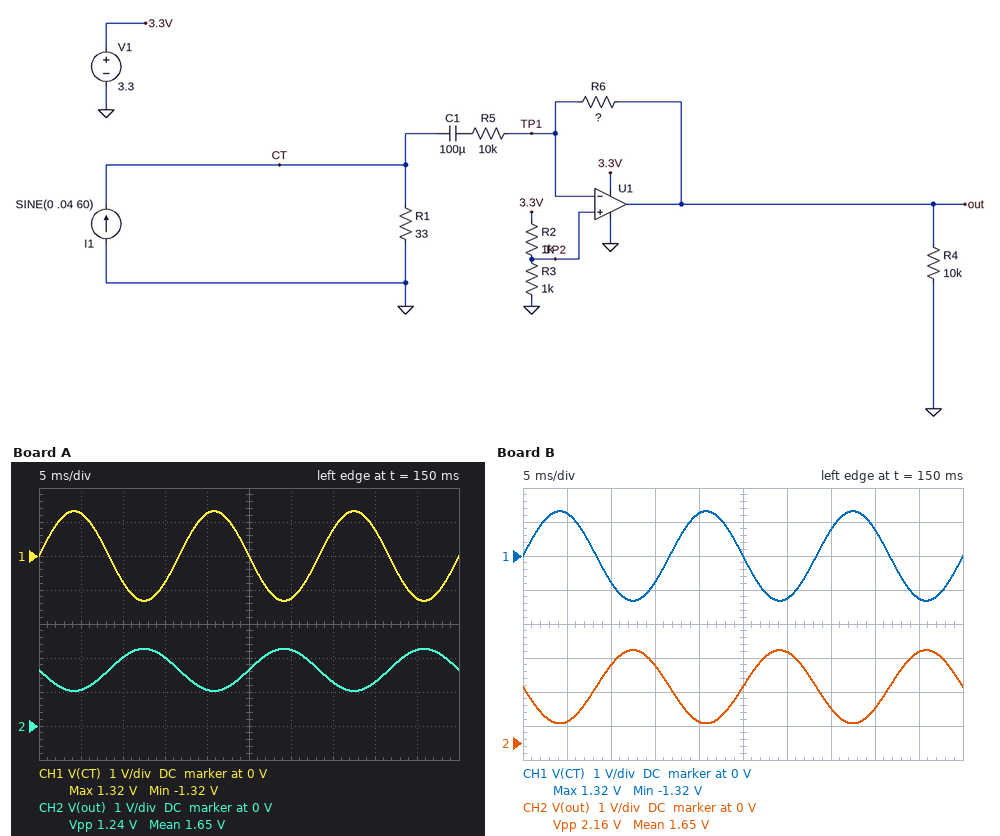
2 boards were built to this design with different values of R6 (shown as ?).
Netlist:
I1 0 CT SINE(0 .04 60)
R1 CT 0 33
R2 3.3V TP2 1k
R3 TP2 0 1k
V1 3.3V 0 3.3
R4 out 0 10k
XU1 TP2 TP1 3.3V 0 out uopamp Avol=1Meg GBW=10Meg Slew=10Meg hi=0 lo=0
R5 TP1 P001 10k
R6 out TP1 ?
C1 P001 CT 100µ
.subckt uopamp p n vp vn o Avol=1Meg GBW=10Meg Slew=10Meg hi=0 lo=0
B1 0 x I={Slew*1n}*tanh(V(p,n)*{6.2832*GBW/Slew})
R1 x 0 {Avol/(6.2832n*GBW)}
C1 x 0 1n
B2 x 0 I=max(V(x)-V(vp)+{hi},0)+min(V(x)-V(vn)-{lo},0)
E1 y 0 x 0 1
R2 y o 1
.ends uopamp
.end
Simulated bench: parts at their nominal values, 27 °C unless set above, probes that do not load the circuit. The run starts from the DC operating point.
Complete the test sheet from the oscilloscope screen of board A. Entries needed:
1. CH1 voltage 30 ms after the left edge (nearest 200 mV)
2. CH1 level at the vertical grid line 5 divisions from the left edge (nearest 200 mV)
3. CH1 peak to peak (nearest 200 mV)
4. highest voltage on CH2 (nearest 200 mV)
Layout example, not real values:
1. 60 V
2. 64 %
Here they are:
1. -1.2 V
2. 0 V
3. 2.6 V
4. 2.2 V
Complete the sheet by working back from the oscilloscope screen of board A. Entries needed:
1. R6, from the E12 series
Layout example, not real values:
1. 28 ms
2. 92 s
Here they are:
1. 4.7 kΩ
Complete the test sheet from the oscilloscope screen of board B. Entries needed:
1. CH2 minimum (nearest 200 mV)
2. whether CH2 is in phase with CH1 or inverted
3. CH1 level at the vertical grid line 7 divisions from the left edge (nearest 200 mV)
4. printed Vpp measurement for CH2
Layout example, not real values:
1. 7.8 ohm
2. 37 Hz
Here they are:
1. 600 mV
2. inverted
3. 800 mV
4. 2.16 V
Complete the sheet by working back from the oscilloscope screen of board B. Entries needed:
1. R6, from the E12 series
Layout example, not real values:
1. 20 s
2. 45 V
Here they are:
1. 8.2 kΩ
